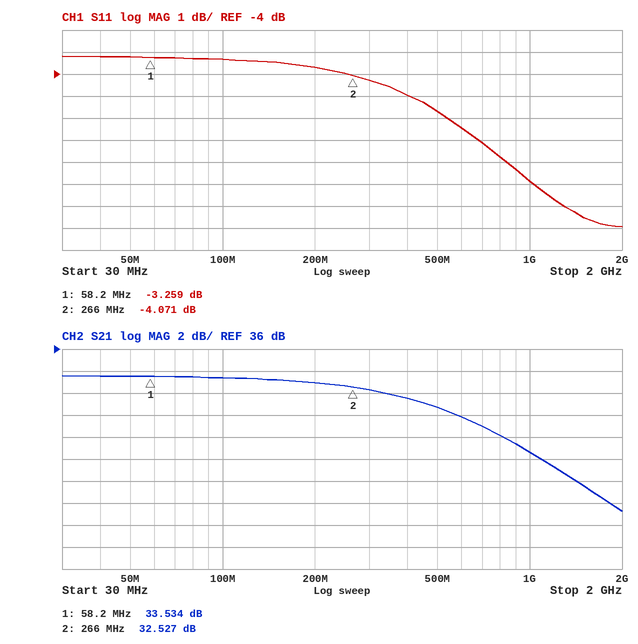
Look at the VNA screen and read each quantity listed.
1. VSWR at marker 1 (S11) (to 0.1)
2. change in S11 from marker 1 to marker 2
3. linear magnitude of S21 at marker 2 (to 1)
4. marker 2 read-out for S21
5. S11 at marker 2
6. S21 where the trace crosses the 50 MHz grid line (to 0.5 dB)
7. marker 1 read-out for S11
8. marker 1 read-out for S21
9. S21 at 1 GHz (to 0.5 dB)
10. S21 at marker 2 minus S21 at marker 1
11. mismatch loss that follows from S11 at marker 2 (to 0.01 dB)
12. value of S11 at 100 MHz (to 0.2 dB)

5.4
-0.812 dB
42
32.527 dB
-4.071 dB
33.5 dB
-3.259 dB
33.534 dB
26.5 dB
-1.007 dB
2.16 dB
-3.4 dB
